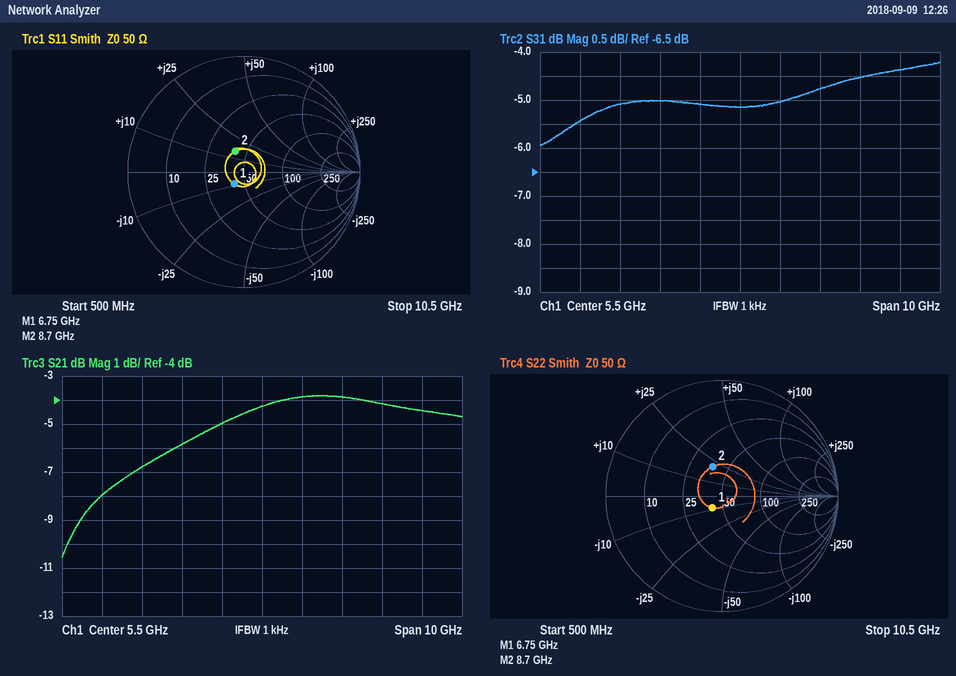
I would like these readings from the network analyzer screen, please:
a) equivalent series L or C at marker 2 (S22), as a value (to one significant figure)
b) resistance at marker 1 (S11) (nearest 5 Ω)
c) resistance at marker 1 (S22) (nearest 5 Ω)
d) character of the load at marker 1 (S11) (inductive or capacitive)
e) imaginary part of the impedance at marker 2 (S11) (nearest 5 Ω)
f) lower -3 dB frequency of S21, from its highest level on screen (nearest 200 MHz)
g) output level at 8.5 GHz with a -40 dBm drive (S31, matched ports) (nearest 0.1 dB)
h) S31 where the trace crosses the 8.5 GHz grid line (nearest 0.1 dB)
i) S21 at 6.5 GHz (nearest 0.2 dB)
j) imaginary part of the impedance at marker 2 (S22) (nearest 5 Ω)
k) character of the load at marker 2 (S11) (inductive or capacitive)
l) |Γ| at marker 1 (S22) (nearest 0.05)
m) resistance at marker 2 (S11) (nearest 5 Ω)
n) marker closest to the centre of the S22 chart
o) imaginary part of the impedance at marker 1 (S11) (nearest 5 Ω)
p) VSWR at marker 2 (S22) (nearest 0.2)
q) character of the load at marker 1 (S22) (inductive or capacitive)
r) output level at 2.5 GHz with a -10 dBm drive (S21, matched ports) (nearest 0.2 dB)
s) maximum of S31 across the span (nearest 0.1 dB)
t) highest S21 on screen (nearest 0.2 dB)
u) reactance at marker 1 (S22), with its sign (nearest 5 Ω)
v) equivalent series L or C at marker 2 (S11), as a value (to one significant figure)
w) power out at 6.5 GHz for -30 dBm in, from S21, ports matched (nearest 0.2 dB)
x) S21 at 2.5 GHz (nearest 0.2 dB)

400 pH
40 Ω
40 Ω
capacitive
+15 Ω
2.4 GHz
-44.5 dBm
-4.5 dB
-3.8 dB
+20 Ω
inductive
0.15
40 Ω
marker 1
-10 Ω
1.8
capacitive
-16.8 dBm
-4.2 dB
-3.8 dB
-10 Ω
300 pH
-33.8 dBm
-6.8 dB
